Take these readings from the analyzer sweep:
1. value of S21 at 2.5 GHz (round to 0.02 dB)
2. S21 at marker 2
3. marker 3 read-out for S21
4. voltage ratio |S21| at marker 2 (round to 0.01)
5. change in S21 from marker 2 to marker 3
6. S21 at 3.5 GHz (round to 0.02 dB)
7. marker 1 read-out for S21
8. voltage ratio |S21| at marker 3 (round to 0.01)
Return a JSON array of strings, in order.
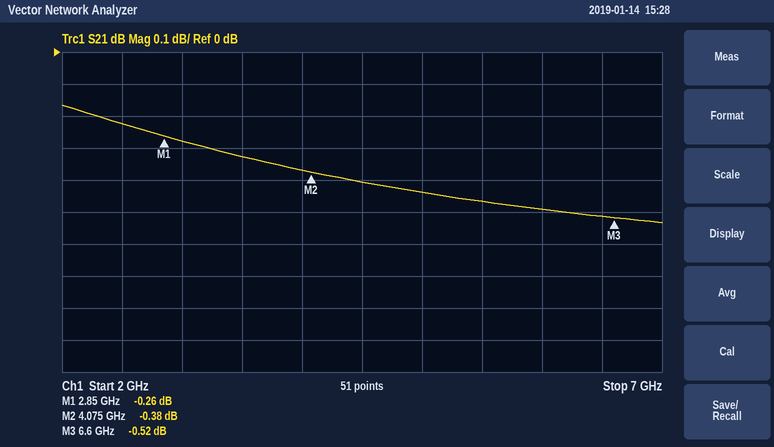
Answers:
["-0.22 dB", "-0.38 dB", "-0.52 dB", "0.96", "-0.14 dB", "-0.32 dB", "-0.26 dB", "0.94"]
